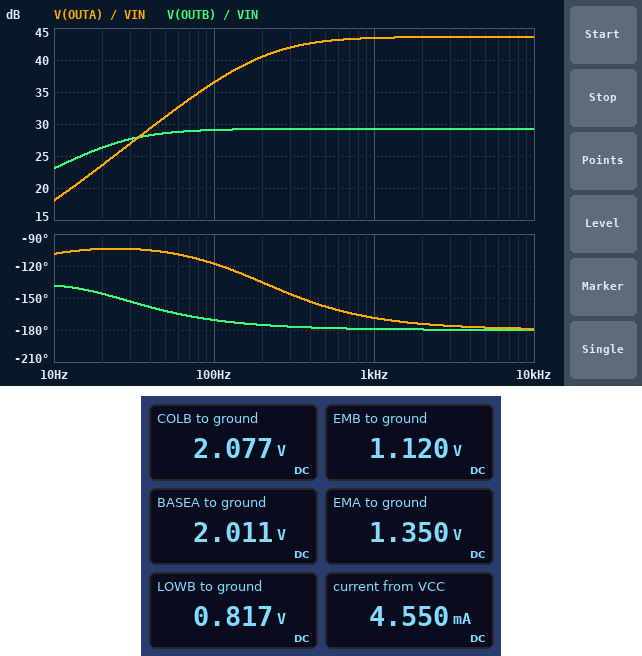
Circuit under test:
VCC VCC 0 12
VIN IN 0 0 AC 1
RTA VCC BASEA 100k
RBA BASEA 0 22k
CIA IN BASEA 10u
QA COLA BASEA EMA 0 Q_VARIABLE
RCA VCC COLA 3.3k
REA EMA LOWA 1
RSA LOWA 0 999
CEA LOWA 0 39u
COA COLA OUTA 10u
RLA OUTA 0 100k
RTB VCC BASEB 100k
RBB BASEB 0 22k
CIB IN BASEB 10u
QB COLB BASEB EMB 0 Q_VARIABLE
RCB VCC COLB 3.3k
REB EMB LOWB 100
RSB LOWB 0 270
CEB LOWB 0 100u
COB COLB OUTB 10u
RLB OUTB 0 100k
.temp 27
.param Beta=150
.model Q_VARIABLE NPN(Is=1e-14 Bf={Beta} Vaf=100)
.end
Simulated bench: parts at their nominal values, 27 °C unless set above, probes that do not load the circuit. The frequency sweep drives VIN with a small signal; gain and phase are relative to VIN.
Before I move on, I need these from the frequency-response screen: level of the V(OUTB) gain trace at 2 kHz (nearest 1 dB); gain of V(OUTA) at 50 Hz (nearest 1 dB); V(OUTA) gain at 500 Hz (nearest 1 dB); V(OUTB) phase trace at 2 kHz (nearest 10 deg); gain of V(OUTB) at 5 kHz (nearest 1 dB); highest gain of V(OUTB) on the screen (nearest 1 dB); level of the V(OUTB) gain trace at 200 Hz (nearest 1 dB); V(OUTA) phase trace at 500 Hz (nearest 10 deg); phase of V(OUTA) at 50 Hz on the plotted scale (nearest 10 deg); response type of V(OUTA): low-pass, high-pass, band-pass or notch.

29 dB
31 dB
43 dB
-180 deg
29 dB
29 dB
29 dB
-160 deg
-110 deg
high-pass
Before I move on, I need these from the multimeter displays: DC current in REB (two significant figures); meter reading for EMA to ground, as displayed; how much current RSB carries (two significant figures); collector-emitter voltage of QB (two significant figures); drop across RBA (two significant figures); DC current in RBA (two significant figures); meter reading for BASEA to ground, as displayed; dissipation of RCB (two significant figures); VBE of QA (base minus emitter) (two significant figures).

3.0 mA
1.350 V
3.0 mA
960 mV
2.0 V
91 µA
2.011 V
30 mW
660 mV
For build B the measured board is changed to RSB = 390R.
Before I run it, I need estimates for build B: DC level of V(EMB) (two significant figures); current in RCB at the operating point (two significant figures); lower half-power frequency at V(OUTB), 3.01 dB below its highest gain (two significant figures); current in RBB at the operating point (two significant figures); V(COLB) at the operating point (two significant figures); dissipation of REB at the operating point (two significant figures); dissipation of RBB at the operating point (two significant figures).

1.2 V
2.4 mA
18 Hz
85 µA
4.0 V
600 µW
160 µW
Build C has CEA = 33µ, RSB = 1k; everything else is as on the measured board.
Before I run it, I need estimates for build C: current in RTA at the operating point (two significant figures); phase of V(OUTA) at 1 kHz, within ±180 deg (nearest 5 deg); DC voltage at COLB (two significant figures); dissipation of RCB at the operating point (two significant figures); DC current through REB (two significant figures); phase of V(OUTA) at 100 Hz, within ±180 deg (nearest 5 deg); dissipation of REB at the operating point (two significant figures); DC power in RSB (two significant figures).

100 µA
-165 deg
7.9 V
5.0 mW
1.2 mA
-115 deg
150 µW
1.5 mW
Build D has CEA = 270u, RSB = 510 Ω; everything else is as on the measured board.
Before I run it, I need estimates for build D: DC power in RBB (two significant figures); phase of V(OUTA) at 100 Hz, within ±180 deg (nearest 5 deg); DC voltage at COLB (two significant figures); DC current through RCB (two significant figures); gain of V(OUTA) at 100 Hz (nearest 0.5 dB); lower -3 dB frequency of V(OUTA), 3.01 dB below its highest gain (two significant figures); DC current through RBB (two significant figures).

170 µW
-160 deg
5.3 V
2.0 mA
43.0 dB
34 Hz
88 µA
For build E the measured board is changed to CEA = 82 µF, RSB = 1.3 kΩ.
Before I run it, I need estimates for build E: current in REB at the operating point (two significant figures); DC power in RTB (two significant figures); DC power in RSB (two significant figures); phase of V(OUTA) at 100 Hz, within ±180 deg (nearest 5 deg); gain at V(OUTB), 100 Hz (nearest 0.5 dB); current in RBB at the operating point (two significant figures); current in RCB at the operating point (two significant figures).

1.0 mA
990 µW
1.3 mW
-135 deg
28.0 dB
93 µA
990 µA
